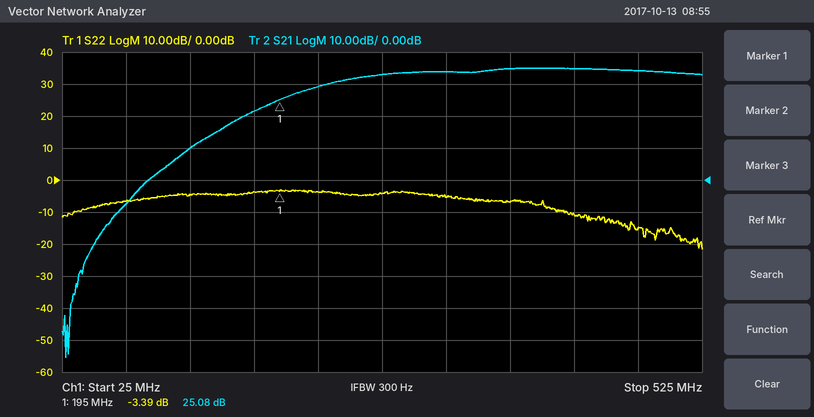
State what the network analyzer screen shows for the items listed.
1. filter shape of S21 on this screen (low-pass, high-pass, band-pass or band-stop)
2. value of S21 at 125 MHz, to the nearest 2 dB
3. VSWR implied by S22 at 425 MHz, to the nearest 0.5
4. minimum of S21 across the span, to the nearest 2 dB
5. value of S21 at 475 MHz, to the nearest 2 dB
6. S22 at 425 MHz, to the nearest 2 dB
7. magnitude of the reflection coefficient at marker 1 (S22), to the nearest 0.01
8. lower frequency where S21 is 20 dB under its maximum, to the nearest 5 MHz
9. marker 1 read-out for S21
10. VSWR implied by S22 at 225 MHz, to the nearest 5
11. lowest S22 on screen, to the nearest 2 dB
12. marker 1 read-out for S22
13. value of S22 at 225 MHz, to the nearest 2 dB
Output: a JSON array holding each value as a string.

["high-pass", "10 dB", "2.0", "-56 dB", "34 dB", "-10 dB", "0.68", "145 MHz", "25.08 dB", "5", "-22 dB", "-3.39 dB", "-4 dB"]
